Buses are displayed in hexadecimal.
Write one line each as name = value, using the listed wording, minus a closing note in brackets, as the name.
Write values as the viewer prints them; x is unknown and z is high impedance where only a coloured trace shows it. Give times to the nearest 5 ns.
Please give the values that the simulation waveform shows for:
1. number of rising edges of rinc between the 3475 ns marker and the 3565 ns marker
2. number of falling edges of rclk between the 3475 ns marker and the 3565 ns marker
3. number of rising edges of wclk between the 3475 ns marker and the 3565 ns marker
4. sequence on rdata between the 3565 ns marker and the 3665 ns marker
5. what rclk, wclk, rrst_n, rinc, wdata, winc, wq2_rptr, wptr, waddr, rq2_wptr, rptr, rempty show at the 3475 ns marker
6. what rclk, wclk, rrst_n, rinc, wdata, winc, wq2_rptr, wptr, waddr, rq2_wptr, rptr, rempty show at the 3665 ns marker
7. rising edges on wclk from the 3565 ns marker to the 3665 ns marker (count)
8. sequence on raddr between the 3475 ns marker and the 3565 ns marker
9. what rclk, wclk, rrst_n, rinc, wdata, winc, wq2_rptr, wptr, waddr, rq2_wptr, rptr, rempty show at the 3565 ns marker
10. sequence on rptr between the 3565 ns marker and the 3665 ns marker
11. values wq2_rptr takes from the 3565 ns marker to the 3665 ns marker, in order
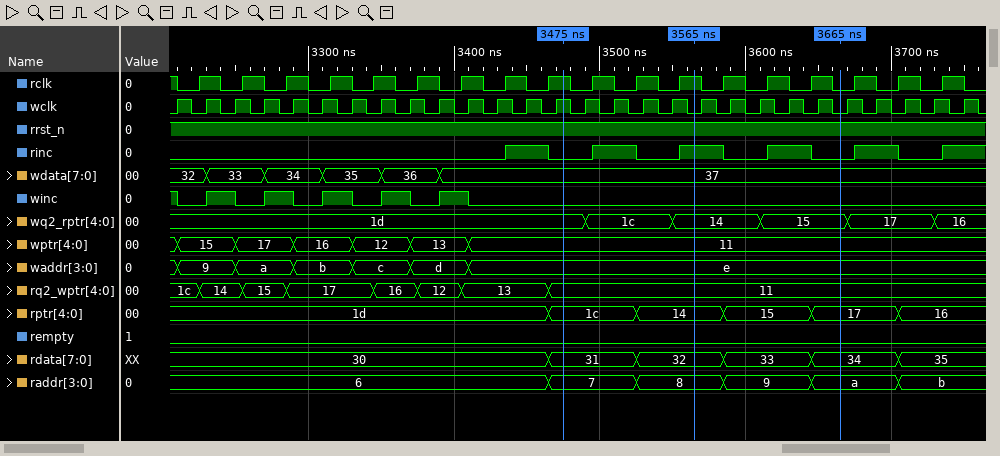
number of rising edges of rinc between the 3475 ns marker and the 3565 ns marker = 2
number of falling edges of rclk between the 3475 ns marker and the 3565 ns marker = 3
number of rising edges of wclk between the 3475 ns marker and the 3565 ns marker = 4
sequence on rdata between the 3565 ns marker and the 3665 ns marker = 32, 33, 34
what rclk, wclk, rrst_n, rinc, wdata, winc, wq2_rptr, wptr, waddr, rq2_wptr, rptr, rempty show at the 3475 ns marker = rclk=1, wclk=1, rrst_n=1, rinc=0, wdata=37, winc=0, wq2_rptr=1d, wptr=11, waddr=e, rq2_wptr=11, rptr=1c, rempty=0
what rclk, wclk, rrst_n, rinc, wdata, winc, wq2_rptr, wptr, waddr, rq2_wptr, rptr, rempty show at the 3665 ns marker = rclk=0, wclk=0, rrst_n=1, rinc=0, wdata=37, winc=0, wq2_rptr=15, wptr=11, waddr=e, rq2_wptr=11, rptr=17, rempty=0
rising edges on wclk from the 3565 ns marker to the 3665 ns marker = 5
sequence on raddr between the 3475 ns marker and the 3565 ns marker = 7, 8
what rclk, wclk, rrst_n, rinc, wdata, winc, wq2_rptr, wptr, waddr, rq2_wptr, rptr, rempty show at the 3565 ns marker = rclk=1, wclk=0, rrst_n=1, rinc=1, wdata=37, winc=0, wq2_rptr=14, wptr=11, waddr=e, rq2_wptr=11, rptr=14, rempty=0
sequence on rptr between the 3565 ns marker and the 3665 ns marker = 14, 15, 17
values wq2_rptr takes from the 3565 ns marker to the 3665 ns marker, in order = 14, 15
